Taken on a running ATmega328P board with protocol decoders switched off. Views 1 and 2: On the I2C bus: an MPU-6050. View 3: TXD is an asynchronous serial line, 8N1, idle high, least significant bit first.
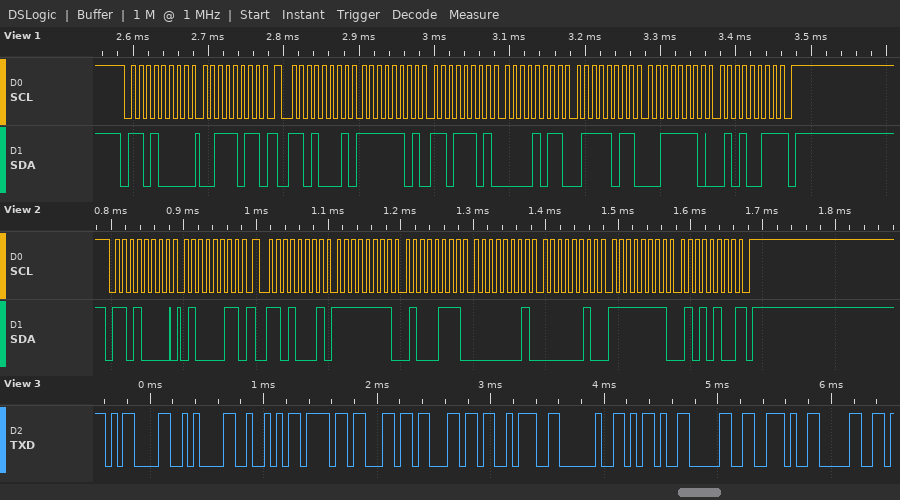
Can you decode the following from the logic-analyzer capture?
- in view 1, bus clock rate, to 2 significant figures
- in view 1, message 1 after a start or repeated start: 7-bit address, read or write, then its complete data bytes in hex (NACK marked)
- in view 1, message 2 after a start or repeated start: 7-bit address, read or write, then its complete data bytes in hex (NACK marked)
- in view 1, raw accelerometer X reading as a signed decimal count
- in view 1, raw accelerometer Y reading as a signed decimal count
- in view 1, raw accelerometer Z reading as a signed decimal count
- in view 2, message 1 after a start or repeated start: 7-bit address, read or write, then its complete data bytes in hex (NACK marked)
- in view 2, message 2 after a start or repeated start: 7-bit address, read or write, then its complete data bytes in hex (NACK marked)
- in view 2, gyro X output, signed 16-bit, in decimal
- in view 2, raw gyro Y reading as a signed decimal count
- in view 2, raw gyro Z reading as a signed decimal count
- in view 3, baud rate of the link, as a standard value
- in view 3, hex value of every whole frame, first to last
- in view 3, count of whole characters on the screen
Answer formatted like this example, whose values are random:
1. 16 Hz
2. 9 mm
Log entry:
1. 100 kHz
2. 0x68 write: 3B
3. 0x68 read: FD DD 0B 7B 3E 53 NACK
4. -547
5. 2939
6. 15955
7. 0x68 write: 43
8. 0x68 read: FF 47 01 02 FF 54 NACK
9. -185
10. 258
11. -172
12. 19200 baud
13. 0x0D 0x0A 0x52 0x6F 0x6C 0x6C 0x3A 0x20 0x2D 0x30 0x2E 0x30
14. 12
